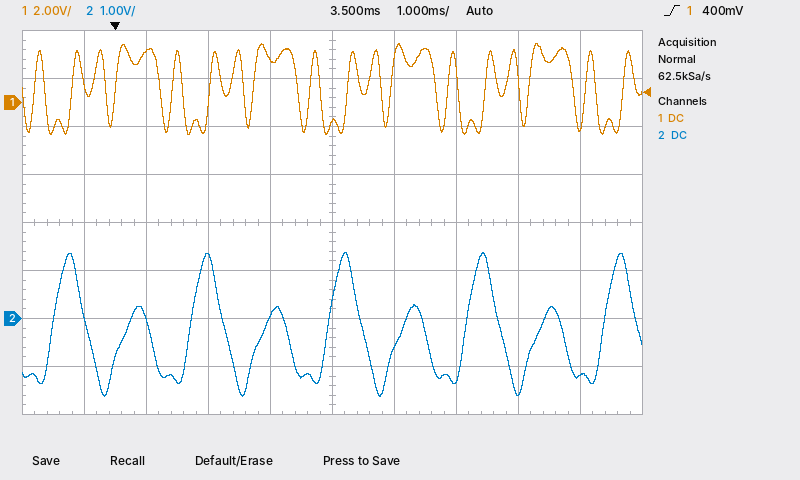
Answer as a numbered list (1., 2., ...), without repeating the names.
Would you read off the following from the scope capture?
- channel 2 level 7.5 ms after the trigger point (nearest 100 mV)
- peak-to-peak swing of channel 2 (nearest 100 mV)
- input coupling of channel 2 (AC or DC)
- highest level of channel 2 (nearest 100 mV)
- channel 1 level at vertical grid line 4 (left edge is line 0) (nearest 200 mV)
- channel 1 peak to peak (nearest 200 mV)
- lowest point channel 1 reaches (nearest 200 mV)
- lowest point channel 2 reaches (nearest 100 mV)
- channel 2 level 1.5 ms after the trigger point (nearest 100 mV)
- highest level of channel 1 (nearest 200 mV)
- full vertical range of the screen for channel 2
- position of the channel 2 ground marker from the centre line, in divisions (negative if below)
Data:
1. -1.2 V
2. 3.0 V
3. DC
4. 1.4 V
5. 1.8 V
6. 3.8 V
7. -1.4 V
8. -1.6 V
9. 1.3 V
10. 2.4 V
11. 8 V
12. -2.0 div
